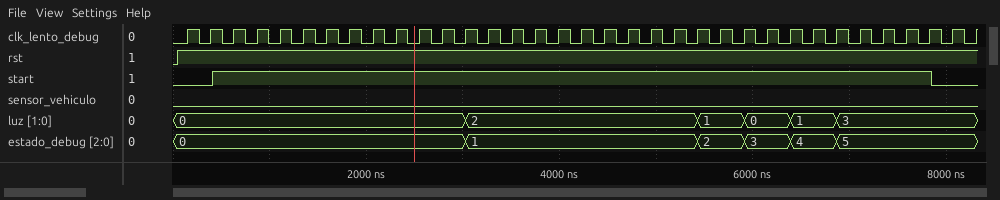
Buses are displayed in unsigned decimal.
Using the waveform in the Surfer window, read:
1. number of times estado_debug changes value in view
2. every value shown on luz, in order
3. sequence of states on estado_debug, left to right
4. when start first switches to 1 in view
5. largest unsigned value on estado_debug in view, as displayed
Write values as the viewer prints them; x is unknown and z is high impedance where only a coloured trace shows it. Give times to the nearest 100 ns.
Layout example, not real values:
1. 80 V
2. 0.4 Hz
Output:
1. 5
2. 0, 2, 1, 0, 1, 3
3. 0, 1, 2, 3, 4, 5
4. 400 ns
5. 5
